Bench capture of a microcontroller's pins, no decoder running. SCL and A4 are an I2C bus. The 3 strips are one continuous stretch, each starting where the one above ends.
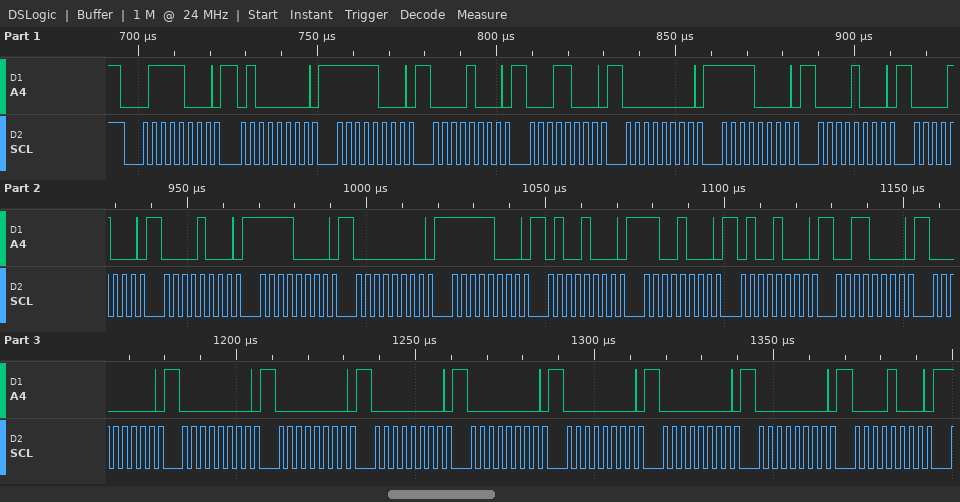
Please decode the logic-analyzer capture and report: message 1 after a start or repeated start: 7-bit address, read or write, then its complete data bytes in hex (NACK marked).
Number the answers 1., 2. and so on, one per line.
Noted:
1. 0x3C write: 40 F8 08 18 00 F0 08 08 08 F0 00 F8 48 C8 48 30 00 00 00 00 00 00 00 00 08
